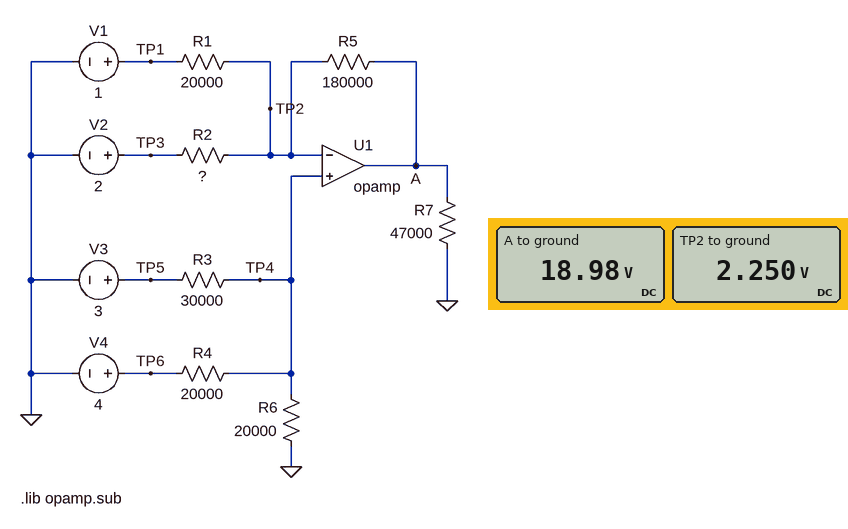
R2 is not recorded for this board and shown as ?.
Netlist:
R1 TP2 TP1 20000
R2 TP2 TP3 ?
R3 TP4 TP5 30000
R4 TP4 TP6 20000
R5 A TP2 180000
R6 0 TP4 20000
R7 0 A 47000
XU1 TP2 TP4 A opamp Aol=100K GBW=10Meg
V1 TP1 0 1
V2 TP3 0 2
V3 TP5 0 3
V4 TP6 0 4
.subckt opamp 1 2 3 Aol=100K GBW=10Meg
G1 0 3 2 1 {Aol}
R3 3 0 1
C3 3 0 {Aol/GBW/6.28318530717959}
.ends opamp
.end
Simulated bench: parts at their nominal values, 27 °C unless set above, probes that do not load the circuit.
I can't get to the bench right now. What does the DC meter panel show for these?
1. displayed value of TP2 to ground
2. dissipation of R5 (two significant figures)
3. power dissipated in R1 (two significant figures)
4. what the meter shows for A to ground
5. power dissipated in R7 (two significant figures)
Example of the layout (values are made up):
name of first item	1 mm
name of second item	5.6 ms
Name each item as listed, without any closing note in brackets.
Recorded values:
displayed value of TP2 to ground	2.250 V
dissipation of R5	1.6 mW
power dissipated in R1	78 µW
what the meter shows for A to ground	18.98 V
power dissipated in R7	7.7 mW
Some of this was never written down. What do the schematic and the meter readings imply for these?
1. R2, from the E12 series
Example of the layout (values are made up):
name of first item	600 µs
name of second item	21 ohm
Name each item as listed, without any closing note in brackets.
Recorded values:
R2, from the E12 series	8.2 kΩ
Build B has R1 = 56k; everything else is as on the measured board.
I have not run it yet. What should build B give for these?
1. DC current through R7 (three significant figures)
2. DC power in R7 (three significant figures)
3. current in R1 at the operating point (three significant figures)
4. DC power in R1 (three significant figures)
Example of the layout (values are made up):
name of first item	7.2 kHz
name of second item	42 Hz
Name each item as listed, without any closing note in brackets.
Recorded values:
DC current through R7	250 µA
DC power in R7	2.94 mW
current in R1 at the operating point	22.3 µA
DC power in R1	27.9 µW
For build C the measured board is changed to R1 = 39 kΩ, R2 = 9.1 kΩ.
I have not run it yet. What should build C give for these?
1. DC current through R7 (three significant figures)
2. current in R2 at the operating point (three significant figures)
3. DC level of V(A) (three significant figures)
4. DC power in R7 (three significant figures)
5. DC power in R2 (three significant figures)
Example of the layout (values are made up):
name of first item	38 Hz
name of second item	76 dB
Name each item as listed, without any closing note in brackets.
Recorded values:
DC current through R7	276 µA
current in R2 at the operating point	27.5 µA
DC level of V(A)	13.0 V
DC power in R7	3.57 mW
DC power in R2	6.86 µW
